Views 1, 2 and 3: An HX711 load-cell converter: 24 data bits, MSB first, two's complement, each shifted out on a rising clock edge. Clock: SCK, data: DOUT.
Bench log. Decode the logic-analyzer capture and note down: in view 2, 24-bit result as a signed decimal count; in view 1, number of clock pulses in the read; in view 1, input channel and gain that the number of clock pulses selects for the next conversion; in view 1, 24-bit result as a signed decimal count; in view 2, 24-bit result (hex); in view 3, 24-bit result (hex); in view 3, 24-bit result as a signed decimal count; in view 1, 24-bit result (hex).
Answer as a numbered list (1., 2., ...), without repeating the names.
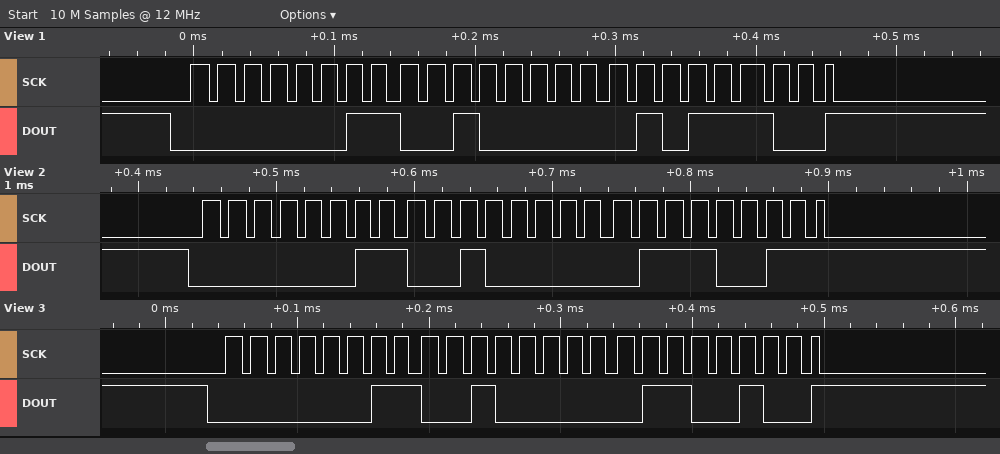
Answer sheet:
1. 204915
2. 25
3. channel A, gain 128
4. 204892
5. 0x032073
6. 0x032064
7. 204900
8. 0x03205C
